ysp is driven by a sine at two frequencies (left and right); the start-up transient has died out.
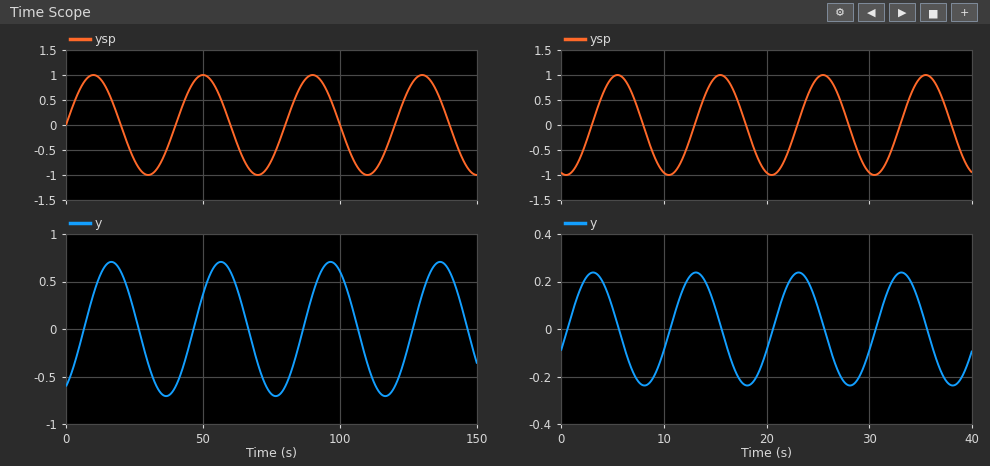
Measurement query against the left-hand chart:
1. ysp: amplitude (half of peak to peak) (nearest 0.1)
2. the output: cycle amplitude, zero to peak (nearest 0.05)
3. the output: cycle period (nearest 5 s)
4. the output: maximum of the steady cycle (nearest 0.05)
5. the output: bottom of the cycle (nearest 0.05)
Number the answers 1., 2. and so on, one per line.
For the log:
1. 1.0
2. 0.70
3. 40 s
4. 0.70
5. -0.70
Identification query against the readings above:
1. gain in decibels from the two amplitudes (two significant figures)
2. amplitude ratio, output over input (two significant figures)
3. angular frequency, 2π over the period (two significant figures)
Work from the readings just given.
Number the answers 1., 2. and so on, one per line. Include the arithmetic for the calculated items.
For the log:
1. 20 log10(0.7 / 1) = -3.1 dB
2. 0.7 / 1 = 0.70
3. 2π / 40 = 0.16 rad/s
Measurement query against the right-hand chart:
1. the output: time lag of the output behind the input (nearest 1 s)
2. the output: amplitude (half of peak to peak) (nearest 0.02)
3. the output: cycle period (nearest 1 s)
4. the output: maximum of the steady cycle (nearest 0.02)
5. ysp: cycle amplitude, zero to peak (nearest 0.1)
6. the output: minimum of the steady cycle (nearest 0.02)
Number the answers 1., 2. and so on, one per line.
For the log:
1. 8 s
2. 0.24
3. 10 s
4. 0.24
5. 1.0
6. -0.24
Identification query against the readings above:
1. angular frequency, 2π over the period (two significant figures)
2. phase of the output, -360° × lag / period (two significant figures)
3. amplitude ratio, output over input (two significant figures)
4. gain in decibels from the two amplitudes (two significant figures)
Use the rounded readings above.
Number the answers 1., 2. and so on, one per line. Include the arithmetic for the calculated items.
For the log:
1. 2π / 10 = 0.63 rad/s
2. -360 × 8 / 10 = -290°
3. 0.24 / 1 = 0.24
4. 20 log10(0.24 / 1) = -12 dB
